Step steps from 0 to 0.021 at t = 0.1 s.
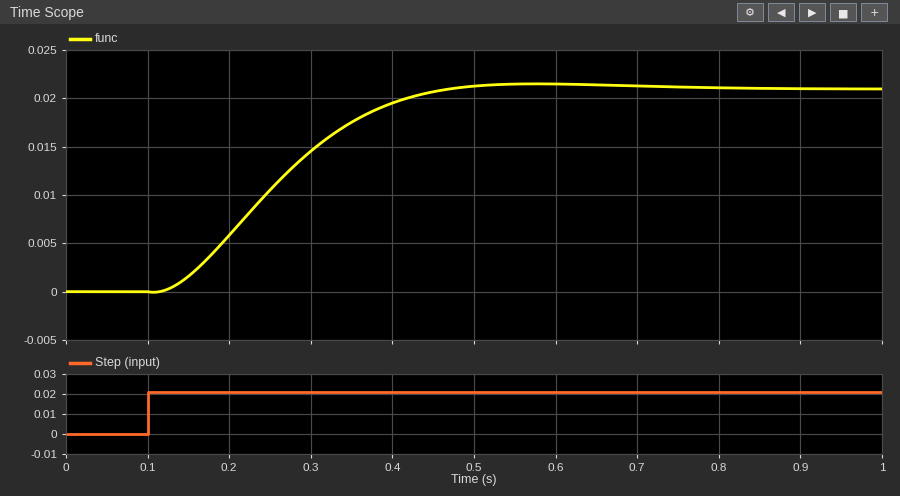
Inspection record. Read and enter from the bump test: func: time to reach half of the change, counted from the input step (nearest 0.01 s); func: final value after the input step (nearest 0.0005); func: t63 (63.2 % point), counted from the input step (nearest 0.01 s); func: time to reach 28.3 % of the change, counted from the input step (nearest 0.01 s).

0.15 s
0.0210
0.18 s
0.10 s
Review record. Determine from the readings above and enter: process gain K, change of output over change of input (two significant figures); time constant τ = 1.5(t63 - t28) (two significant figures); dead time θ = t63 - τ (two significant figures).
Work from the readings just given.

1.0
0.12 s
0.060 s
